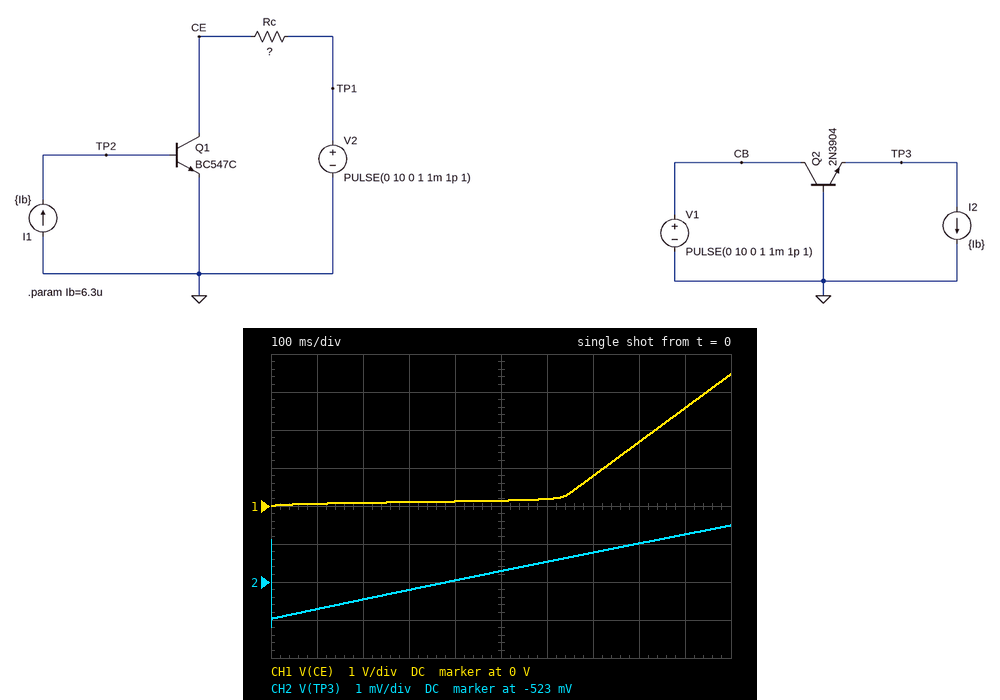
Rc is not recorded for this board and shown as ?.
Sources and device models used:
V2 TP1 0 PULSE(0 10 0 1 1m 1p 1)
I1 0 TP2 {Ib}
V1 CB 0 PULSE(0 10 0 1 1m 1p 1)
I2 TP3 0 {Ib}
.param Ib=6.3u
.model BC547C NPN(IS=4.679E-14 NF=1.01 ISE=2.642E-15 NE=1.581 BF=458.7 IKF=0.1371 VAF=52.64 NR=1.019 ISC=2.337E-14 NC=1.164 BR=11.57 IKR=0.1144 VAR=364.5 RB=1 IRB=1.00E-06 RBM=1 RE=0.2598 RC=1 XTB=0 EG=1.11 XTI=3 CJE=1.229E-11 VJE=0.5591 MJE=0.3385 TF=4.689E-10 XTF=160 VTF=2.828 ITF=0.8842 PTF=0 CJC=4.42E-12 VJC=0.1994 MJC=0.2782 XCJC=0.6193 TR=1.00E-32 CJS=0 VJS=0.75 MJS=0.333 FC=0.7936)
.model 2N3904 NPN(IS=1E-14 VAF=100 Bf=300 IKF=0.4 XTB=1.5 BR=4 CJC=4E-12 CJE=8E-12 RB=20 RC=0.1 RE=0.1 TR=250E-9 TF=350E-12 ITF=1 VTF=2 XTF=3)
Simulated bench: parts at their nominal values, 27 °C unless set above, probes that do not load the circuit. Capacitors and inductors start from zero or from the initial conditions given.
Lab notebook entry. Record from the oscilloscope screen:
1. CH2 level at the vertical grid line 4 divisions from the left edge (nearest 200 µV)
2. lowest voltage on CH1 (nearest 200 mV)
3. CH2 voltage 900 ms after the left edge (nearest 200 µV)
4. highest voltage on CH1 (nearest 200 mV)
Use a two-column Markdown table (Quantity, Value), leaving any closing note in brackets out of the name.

| Quantity | Value |
|---|---|
| CH2 level at the vertical grid line 4 divisions from the left edge | -523.0 mV |
| lowest voltage on CH1 | 0 V |
| CH2 voltage 900 ms after the left edge | -521.8 mV |
| highest voltage on CH1 | 3.4 V |
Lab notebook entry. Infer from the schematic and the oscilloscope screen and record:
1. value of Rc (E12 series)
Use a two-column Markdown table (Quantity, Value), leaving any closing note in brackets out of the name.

| Quantity | Value |
|---|---|
| value of Rc | 2.2 kΩ |
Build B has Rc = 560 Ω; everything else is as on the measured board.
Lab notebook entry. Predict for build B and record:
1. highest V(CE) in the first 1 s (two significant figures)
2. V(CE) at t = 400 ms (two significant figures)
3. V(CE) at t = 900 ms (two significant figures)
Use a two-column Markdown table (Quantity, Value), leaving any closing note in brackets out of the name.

| Quantity | Value |
|---|---|
| highest V(CE) in the first 1 s | 8.2 V |
| V(CE) at t = 400 ms | 2.4 V |
| V(CE) at t = 900 ms | 7.2 V |
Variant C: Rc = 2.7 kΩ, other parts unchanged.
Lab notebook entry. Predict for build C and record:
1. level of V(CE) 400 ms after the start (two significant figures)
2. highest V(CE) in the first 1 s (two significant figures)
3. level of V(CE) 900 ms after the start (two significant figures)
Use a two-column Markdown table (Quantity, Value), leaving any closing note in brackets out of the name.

| Quantity | Value |
|---|---|
| level of V(CE) 400 ms after the start | 110 mV |
| highest V(CE) in the first 1 s | 2.2 V |
| level of V(CE) 900 ms after the start | 1.3 V |
